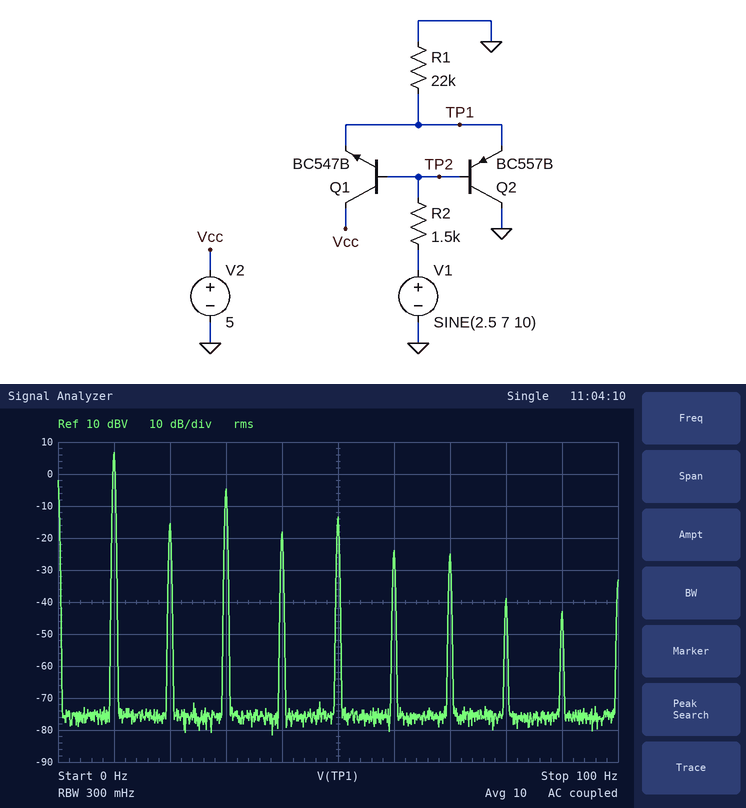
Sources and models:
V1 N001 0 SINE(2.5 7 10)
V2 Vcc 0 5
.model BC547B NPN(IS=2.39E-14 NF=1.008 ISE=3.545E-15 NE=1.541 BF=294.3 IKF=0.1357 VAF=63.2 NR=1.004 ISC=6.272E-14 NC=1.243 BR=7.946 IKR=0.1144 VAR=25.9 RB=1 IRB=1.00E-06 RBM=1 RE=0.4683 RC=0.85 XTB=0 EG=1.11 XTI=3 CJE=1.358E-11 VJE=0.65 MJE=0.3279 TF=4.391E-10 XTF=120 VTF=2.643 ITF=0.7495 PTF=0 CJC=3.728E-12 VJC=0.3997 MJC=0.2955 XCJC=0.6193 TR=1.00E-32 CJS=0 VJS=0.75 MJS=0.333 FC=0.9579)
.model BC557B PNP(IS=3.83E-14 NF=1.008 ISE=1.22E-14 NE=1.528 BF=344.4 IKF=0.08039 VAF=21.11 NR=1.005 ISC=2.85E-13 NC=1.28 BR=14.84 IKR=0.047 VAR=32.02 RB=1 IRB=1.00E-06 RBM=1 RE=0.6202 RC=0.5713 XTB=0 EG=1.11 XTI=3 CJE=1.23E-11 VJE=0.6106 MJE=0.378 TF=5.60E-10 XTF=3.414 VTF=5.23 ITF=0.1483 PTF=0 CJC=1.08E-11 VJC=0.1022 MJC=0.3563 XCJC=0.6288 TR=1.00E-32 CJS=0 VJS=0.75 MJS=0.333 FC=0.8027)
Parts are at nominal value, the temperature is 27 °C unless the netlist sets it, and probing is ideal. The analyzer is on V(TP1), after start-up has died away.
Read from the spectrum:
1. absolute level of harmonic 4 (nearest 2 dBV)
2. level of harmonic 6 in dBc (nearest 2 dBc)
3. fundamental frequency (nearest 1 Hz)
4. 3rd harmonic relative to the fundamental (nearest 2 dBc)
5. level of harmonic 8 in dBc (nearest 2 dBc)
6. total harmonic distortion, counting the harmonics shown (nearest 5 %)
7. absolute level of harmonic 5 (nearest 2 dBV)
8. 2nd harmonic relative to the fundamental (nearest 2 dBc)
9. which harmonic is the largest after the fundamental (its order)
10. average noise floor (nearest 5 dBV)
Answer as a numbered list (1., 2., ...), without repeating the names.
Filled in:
1. -18 dBV
2. -30 dBc
3. 10 Hz
4. -12 dBc
5. -46 dBc
6. 30 %
7. -14 dBV
8. -22 dBc
9. 3
10. -75 dBV
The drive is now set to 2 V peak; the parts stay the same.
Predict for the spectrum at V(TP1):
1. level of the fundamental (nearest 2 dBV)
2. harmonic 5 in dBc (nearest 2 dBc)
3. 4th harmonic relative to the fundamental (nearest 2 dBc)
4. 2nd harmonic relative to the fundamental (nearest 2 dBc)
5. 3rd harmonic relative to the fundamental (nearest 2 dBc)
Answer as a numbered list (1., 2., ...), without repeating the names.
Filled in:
1. 2 dBV
2. -54 dBc
3. -50 dBc
4. -40 dBc
5. -46 dBc
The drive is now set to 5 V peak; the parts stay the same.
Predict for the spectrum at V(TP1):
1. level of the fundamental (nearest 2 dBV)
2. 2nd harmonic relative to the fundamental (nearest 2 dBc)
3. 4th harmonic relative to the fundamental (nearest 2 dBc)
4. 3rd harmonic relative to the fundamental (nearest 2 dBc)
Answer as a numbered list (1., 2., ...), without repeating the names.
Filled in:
1. 6 dBV
2. -20 dBc
3. -26 dBc
4. -14 dBc
